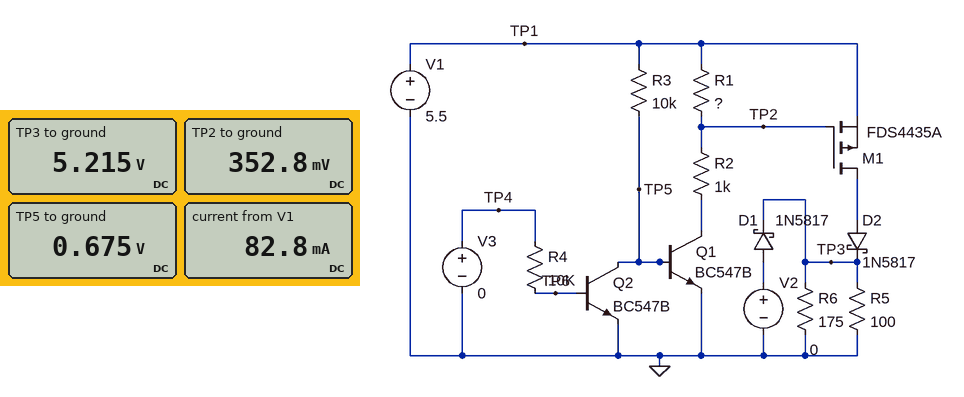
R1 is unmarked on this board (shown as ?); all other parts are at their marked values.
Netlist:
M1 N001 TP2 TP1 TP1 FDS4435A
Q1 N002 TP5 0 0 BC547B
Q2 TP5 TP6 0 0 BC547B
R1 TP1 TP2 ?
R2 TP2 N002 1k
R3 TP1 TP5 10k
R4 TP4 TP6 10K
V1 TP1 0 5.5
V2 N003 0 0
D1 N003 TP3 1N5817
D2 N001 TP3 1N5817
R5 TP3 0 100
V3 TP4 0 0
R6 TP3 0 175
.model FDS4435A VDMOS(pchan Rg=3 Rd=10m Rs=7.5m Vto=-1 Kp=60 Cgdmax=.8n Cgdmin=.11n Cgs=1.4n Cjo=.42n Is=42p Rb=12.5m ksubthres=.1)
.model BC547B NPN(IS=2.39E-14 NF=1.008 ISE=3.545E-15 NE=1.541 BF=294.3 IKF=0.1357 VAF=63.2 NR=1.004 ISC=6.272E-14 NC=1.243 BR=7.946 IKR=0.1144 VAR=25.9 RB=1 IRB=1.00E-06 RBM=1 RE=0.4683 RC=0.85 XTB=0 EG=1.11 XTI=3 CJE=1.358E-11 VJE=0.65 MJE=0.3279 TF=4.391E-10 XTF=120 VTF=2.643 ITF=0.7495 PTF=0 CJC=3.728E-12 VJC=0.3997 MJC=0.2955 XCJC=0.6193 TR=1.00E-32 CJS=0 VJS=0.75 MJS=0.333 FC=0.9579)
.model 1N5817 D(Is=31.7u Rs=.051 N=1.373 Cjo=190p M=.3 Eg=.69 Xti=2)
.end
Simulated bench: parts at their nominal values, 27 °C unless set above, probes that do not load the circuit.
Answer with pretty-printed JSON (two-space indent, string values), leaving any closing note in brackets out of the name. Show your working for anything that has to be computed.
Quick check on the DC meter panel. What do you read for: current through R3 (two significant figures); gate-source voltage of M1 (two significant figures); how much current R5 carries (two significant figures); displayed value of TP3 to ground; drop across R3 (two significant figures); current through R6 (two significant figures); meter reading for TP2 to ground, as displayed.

{
  "current through R3": "(5.5 V - 675 mV) / 10 kΩ = 480 µA",
  "gate-source voltage of M1": "352.8 mV - 5.5 V = -5.1 V",
  "how much current R5 carries": "(5.215 V) / 100 Ω = 52 mA",
  "displayed value of TP3 to ground": "5.215 V",
  "drop across R3": "5.5 V - 675 mV = 4.8 V",
  "current through R6": "(5.215 V) / 175 Ω = 30 mA",
  "meter reading for TP2 to ground, as displayed": "352.8 mV"
}
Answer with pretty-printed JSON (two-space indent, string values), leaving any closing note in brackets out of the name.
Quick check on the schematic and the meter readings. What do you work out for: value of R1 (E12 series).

{
  "value of R1": "15 kΩ"
}
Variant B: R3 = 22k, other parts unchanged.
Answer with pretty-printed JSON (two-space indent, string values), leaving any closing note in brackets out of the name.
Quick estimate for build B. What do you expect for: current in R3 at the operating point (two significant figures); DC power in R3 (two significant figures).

{
  "current in R3 at the operating point": "220 µA",
  "DC power in R3": "1.1 mW"
}
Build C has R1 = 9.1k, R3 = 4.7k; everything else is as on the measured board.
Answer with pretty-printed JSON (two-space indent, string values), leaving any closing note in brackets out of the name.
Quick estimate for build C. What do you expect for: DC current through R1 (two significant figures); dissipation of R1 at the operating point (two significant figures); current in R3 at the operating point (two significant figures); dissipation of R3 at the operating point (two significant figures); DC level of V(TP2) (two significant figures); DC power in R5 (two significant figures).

{
  "DC current through R1": "540 µA",
  "dissipation of R1 at the operating point": "2.7 mW",
  "current in R3 at the operating point": "1.0 mA",
  "dissipation of R3 at the operating point": "4.9 mW",
  "DC level of V(TP2)": "550 mV",
  "DC power in R5": "270 mW"
}
